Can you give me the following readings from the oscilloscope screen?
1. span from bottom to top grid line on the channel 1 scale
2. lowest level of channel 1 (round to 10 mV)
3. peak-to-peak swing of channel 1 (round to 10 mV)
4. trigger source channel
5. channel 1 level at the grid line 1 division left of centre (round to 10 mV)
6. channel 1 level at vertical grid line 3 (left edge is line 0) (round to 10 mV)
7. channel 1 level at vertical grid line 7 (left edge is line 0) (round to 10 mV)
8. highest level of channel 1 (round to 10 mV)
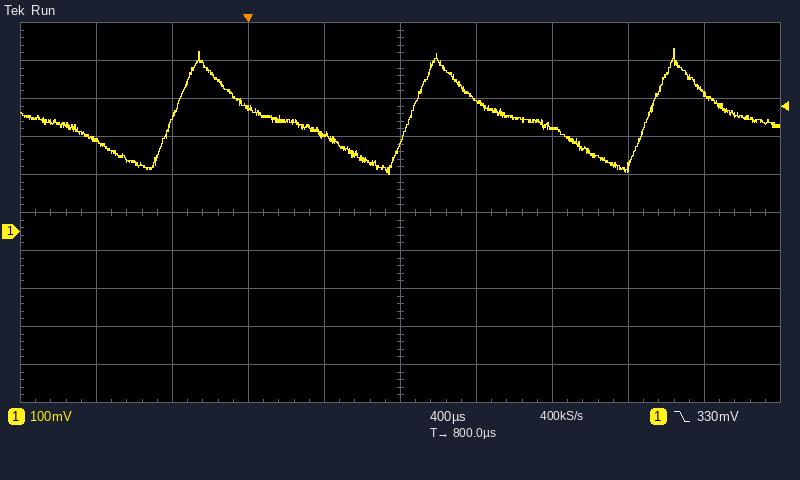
1 V
150 mV
330 mV
channel 1
250 mV
330 mV
280 mV
480 mV
